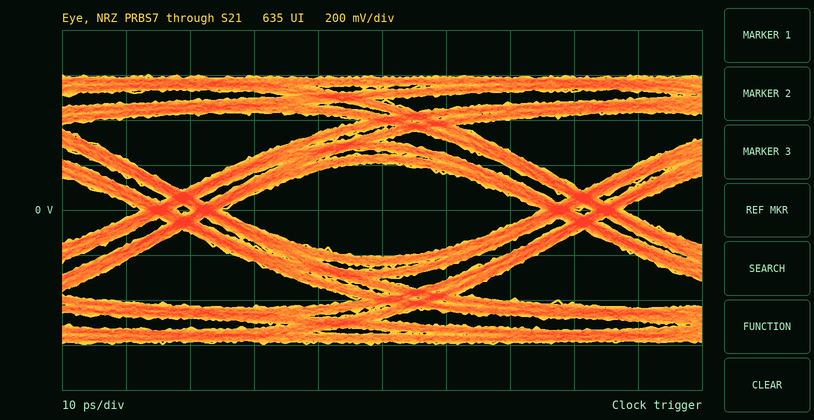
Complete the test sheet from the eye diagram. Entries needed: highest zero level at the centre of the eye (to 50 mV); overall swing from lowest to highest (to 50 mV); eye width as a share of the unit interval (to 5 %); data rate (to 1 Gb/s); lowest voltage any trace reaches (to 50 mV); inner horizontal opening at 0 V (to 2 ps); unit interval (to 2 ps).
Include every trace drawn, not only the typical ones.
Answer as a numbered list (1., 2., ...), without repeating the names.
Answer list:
1. -200 mV
2. 1.20 V
3. 80 %
4. 16 Gb/s
5. -600 mV
6. 50 ps
7. 62 ps
